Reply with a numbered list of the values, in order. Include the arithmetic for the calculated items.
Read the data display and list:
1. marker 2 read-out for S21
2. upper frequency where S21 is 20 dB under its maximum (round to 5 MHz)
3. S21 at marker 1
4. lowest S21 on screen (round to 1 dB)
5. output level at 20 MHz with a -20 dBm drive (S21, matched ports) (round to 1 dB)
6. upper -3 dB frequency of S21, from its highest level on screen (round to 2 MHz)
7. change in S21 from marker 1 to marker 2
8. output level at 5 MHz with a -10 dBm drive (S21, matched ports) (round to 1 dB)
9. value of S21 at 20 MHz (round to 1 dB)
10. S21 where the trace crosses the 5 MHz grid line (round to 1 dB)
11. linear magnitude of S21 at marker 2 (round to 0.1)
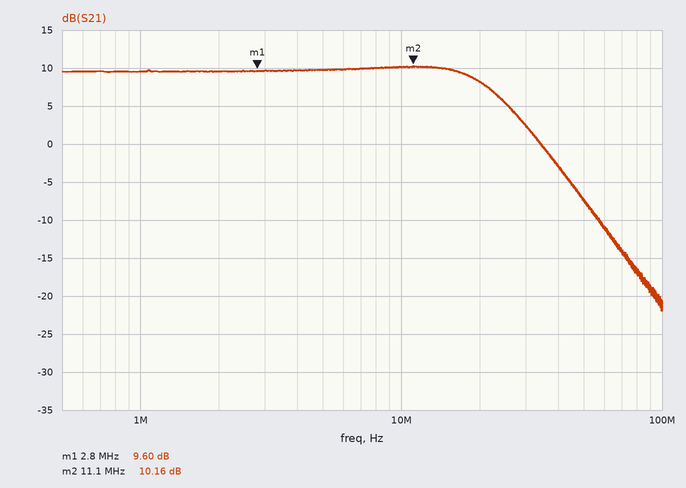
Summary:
1. 10.16 dB
2. 55 MHz
3. 9.60 dB
4. -22 dB
5. -20 dBm + (8 dB) = -12 dBm
6. 22 MHz
7. 10.16 − (9.6) = 0.56 dB
8. -10 dBm + (10 dB) = 0 dBm
9. 8 dB
10. 10 dB
11. 10^(10.16/20) ≈ 3.2
